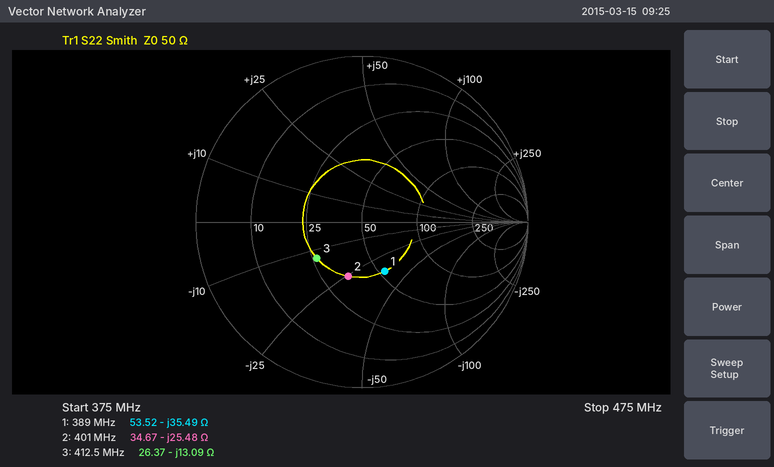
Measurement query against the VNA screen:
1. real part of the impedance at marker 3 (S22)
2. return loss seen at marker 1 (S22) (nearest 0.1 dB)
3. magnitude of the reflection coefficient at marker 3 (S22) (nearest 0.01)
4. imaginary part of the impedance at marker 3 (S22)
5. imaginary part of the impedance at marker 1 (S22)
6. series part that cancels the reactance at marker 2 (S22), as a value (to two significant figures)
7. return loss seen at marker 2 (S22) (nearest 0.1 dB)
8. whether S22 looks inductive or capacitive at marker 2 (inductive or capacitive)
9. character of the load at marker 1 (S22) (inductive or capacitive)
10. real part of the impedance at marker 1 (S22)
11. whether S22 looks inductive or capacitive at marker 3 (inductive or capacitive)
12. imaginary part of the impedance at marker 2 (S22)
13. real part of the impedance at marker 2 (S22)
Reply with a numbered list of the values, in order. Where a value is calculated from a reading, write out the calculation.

1. 26.37 Ω
2. 9.7 dB
3. 0.35
4. -13.09 Ω
5. -35.49 Ω
6. L = 25.48 Ω/(2π × 401 MHz) ≈ 10 nH
7. 9.5 dB
8. capacitive
9. capacitive
10. 53.52 Ω
11. capacitive
12. -25.48 Ω
13. 34.67 Ω
